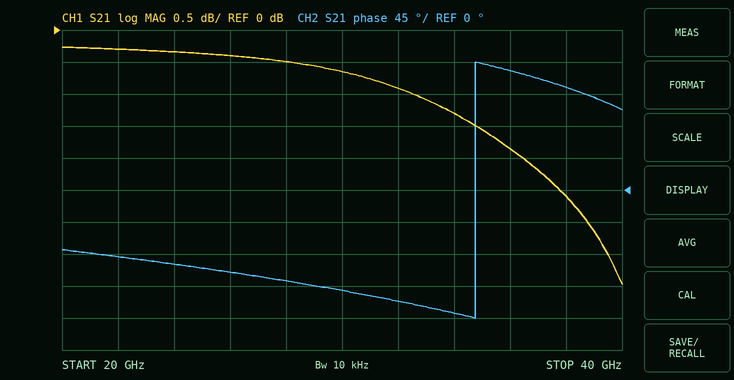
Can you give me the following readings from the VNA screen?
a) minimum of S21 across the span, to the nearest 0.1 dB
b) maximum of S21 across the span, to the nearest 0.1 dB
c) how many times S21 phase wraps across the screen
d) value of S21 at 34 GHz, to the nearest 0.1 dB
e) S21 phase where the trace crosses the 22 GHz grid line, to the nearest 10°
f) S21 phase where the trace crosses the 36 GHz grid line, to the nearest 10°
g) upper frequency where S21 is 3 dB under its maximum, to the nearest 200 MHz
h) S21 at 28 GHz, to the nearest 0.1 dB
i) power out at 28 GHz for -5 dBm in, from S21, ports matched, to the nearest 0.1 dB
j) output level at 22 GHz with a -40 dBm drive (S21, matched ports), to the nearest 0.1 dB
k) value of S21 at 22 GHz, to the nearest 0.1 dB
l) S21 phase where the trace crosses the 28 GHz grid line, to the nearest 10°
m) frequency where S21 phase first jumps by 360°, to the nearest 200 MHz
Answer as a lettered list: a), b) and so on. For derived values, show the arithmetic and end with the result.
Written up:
a) -4.0 dB
b) -0.3 dB
c) 1
d) -1.3 dB
e) -90°
f) 170°
g) 39.2 GHz
h) -0.5 dB
i) -5 dBm + (-0.5 dB) = -5.5 dBm
j) -40 dBm + (-0.3 dB) = -40.3 dBm
k) -0.3 dB
l) -130°
m) 34.8 GHz
